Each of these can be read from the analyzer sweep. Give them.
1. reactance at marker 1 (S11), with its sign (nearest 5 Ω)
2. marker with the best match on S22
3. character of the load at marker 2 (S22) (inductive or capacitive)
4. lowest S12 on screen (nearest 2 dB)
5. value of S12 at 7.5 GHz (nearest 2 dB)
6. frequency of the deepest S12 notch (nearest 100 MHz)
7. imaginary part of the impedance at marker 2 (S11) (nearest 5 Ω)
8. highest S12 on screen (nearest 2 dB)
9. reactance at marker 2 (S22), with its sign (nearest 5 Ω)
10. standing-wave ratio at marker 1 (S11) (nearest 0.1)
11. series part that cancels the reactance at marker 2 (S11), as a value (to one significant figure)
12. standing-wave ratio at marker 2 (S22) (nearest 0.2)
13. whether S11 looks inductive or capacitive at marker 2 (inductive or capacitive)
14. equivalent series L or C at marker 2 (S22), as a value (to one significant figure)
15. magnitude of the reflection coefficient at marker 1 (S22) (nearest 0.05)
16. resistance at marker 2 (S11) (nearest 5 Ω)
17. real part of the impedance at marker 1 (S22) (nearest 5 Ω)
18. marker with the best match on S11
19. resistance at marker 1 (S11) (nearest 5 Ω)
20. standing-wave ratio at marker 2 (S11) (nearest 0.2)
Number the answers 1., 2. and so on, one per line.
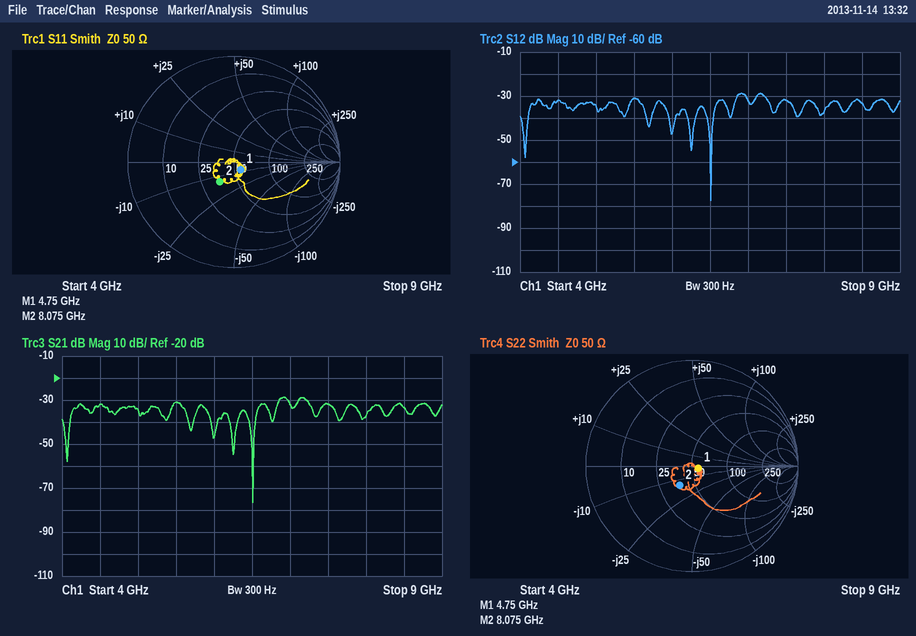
1. -10 Ω
2. marker 1
3. capacitive
4. -78 dB
5. -32 dB
6. 6.5 GHz
7. -15 Ω
8. -28 dB
9. -15 Ω
10. 1.2
11. 300 pH
12. 1.6
13. capacitive
14. 1 pF
15. 0.05
16. 35 Ω
17. 55 Ω
18. marker 1
19. 55 Ω
20. 1.6
